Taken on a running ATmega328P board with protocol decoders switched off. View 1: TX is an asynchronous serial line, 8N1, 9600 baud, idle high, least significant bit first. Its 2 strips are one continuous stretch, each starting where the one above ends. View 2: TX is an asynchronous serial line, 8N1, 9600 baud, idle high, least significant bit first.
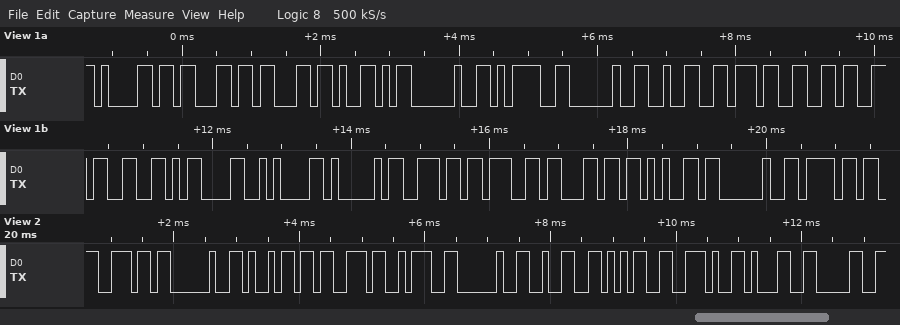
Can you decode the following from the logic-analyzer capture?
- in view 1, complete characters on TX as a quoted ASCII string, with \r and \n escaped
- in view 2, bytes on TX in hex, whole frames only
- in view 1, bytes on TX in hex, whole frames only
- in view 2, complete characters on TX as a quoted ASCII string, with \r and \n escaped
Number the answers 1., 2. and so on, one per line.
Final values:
1. "accY = 2763\r\nAngle o"
2. 6E 20 69 73 3A 20 32 35 2E 31 30
3. 61 63 63 59 20 3D 20 32 37 36 33 0D 0A 41 6E 67 6C 65 20 6F
4. "n is: 25.10"
